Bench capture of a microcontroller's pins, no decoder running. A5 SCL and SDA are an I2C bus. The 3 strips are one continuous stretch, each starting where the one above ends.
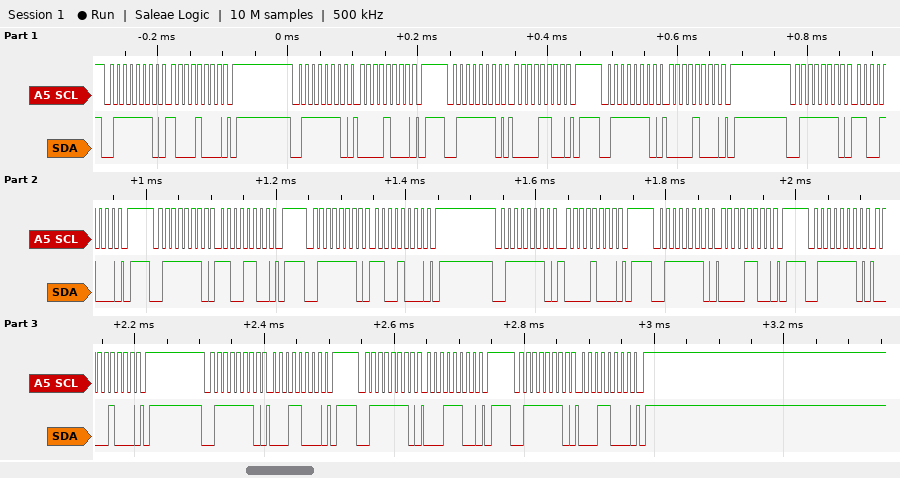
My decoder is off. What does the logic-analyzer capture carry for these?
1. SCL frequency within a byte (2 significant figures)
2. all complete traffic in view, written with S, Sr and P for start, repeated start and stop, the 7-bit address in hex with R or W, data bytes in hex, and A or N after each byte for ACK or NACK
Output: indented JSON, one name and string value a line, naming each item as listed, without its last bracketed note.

{
  "SCL frequency within a byte": "100 kHz",
  "all complete traffic in view, written with S, Sr and P for start, repeated start and stop, the 7-bit address in hex with R or W, data bytes in hex, and A or N after each byte for ACK or NACK": "S 3FW A 88 A P S 3FW A 08 A P S 3FW A 0C A P S 3FW A 08 A P S 3FW A C8 A P S 3FW A CC A P S 3FW A C8 A P S 3FW A 08 A P S 3FW A 0C A P S 3FW A 08 A P S 3FW A 18 A P S 3FW A 1C A P S 3FW A 18 A P"
}
